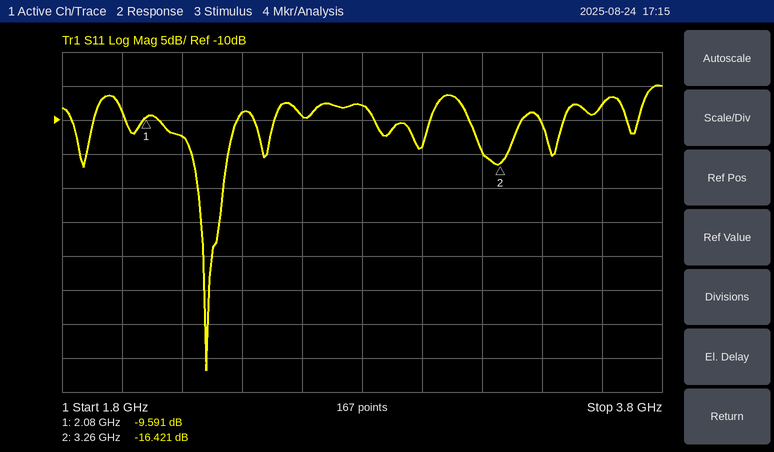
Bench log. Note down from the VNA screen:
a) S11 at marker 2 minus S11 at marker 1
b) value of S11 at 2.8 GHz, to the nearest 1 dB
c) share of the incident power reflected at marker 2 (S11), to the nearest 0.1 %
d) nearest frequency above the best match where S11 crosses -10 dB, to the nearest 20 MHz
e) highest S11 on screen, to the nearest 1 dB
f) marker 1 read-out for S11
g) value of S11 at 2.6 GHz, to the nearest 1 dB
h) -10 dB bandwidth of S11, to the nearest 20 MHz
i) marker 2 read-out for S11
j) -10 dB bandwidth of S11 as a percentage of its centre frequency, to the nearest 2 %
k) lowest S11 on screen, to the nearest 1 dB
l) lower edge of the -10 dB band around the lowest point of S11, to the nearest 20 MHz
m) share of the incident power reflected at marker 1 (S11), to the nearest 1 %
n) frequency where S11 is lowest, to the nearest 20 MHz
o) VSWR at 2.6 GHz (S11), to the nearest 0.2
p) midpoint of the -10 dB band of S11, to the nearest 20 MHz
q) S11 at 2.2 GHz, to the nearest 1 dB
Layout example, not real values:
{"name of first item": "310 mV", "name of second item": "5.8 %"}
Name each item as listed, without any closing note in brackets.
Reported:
{"S11 at marker 2 minus S11 at marker 1": "-6.830 dB", "value of S11 at 2.8 GHz, to the nearest 1 dB": "-8 dB", "share of the incident power reflected at marker 2 (S11), to the nearest 0.1 %": "2.3 %", "nearest frequency above the best match where S11 crosses -10 dB, to the nearest 20 MHz": "2.38 GHz", "highest S11 on screen, to the nearest 1 dB": "-5 dB", "marker 1 read-out for S11": "-9.591 dB", "value of S11 at 2.6 GHz, to the nearest 1 dB": "-9 dB", "-10 dB bandwidth of S11, to the nearest 20 MHz": "260 MHz", "marker 2 read-out for S11": "-16.421 dB", "-10 dB bandwidth of S11 as a percentage of its centre frequency, to the nearest 2 %": "12 %", "lowest S11 on screen, to the nearest 1 dB": "-47 dB", "lower edge of the -10 dB band around the lowest point of S11, to the nearest 20 MHz": "2.12 GHz", "share of the incident power reflected at marker 1 (S11), to the nearest 1 %": "11 %", "frequency where S11 is lowest, to the nearest 20 MHz": "2.28 GHz", "VSWR at 2.6 GHz (S11), to the nearest 0.2": "2.0", "midpoint of the -10 dB band of S11, to the nearest 20 MHz": "2.26 GHz", "S11 at 2.2 GHz, to the nearest 1 dB": "-12 dB"}
